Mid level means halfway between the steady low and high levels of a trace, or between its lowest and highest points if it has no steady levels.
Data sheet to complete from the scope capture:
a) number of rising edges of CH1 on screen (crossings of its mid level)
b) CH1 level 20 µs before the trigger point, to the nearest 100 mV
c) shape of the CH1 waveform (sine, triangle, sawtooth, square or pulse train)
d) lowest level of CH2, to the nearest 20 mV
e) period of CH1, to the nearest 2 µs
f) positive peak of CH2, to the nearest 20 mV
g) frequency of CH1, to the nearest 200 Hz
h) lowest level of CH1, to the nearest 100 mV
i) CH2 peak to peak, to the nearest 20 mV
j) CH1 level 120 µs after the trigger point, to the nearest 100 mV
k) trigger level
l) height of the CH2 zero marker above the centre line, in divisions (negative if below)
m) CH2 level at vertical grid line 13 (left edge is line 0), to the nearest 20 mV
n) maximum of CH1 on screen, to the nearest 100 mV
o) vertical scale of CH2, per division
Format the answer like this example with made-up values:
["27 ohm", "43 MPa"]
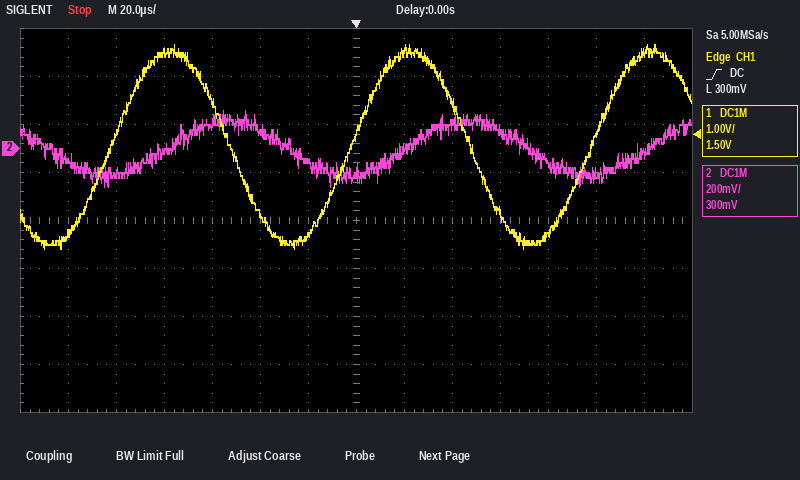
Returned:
["3", "-1.8 V", "sine", "-160 mV", "100 µs", "160 mV", "10.0 kHz", "-2.1 V", "320 mV", "2.0 V", "300 mV", "+1.5 div", "-20 mV", "2.2 V", "200 mV"]
